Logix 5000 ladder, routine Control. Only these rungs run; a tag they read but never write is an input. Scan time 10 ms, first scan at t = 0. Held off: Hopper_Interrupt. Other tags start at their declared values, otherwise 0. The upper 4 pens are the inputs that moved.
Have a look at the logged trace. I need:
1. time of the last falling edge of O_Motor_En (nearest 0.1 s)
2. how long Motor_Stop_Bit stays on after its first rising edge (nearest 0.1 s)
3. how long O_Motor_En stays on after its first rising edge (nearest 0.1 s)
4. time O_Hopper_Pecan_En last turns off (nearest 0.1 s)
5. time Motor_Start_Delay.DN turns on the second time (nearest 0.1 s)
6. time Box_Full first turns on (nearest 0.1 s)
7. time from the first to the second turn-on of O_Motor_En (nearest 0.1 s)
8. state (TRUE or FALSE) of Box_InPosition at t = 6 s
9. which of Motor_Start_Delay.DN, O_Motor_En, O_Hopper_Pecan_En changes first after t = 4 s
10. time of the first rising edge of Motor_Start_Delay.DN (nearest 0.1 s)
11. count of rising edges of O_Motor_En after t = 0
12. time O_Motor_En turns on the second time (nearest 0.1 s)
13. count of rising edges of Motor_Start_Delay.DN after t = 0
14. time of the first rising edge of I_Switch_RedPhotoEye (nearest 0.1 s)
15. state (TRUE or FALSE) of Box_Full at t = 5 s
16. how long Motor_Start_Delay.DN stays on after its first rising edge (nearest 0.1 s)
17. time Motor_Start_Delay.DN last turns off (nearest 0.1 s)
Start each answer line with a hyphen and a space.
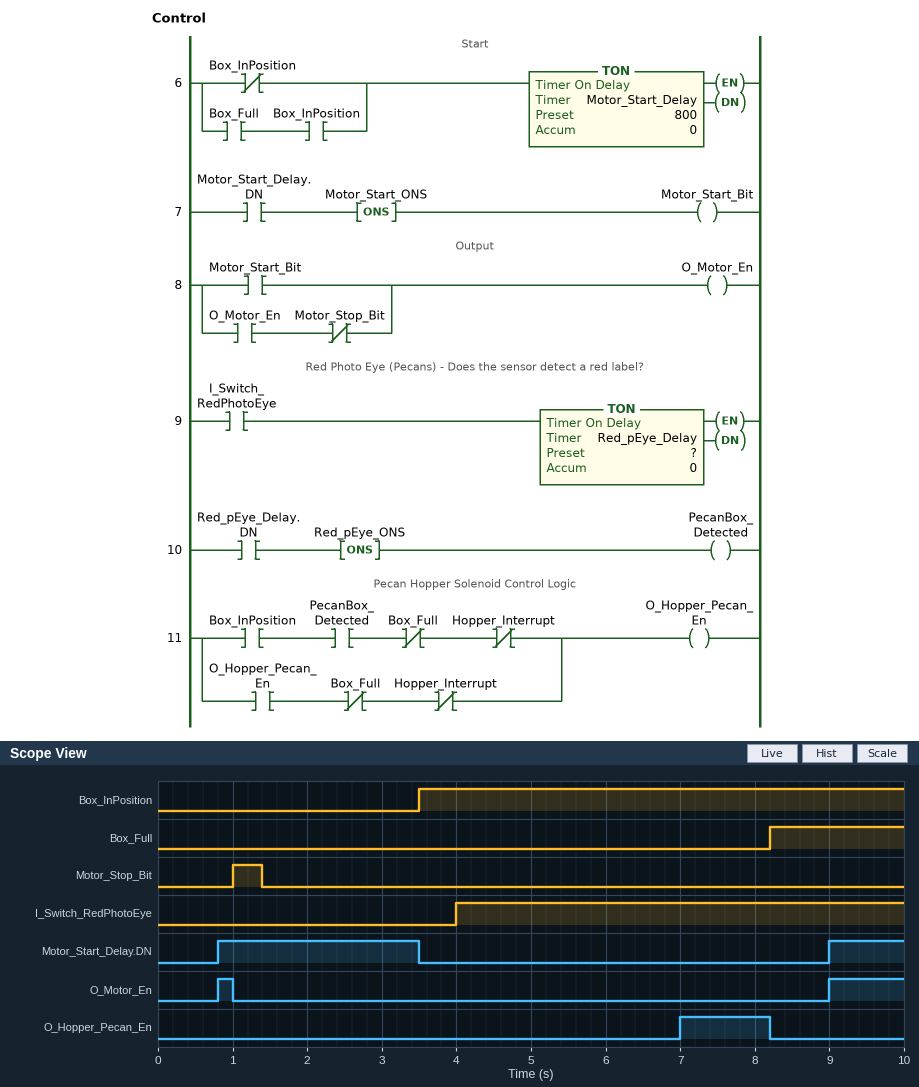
- 1.0 s
- 0.4 s
- 0.2 s
- 8.2 s
- 9.0 s
- 8.2 s
- 8.2 s
- TRUE
- O_Hopper_Pecan_En
- 0.8 s
- 2
- 9.0 s
- 2
- 4.0 s
- FALSE
- 2.7 s
- 3.5 s
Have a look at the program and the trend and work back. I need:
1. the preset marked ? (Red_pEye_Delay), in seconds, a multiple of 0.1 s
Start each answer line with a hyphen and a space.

- 3.0 s
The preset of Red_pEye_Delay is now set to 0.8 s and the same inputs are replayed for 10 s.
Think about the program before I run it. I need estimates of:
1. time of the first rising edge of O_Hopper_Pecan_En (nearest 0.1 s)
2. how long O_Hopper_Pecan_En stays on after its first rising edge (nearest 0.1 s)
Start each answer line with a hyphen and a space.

- 4.8 s
- 3.4 s
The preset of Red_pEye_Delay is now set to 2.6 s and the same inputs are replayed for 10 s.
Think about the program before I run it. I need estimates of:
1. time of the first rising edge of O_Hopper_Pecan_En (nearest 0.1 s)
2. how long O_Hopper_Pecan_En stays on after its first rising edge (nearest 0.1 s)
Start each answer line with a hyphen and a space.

- 6.6 s
- 1.6 s
